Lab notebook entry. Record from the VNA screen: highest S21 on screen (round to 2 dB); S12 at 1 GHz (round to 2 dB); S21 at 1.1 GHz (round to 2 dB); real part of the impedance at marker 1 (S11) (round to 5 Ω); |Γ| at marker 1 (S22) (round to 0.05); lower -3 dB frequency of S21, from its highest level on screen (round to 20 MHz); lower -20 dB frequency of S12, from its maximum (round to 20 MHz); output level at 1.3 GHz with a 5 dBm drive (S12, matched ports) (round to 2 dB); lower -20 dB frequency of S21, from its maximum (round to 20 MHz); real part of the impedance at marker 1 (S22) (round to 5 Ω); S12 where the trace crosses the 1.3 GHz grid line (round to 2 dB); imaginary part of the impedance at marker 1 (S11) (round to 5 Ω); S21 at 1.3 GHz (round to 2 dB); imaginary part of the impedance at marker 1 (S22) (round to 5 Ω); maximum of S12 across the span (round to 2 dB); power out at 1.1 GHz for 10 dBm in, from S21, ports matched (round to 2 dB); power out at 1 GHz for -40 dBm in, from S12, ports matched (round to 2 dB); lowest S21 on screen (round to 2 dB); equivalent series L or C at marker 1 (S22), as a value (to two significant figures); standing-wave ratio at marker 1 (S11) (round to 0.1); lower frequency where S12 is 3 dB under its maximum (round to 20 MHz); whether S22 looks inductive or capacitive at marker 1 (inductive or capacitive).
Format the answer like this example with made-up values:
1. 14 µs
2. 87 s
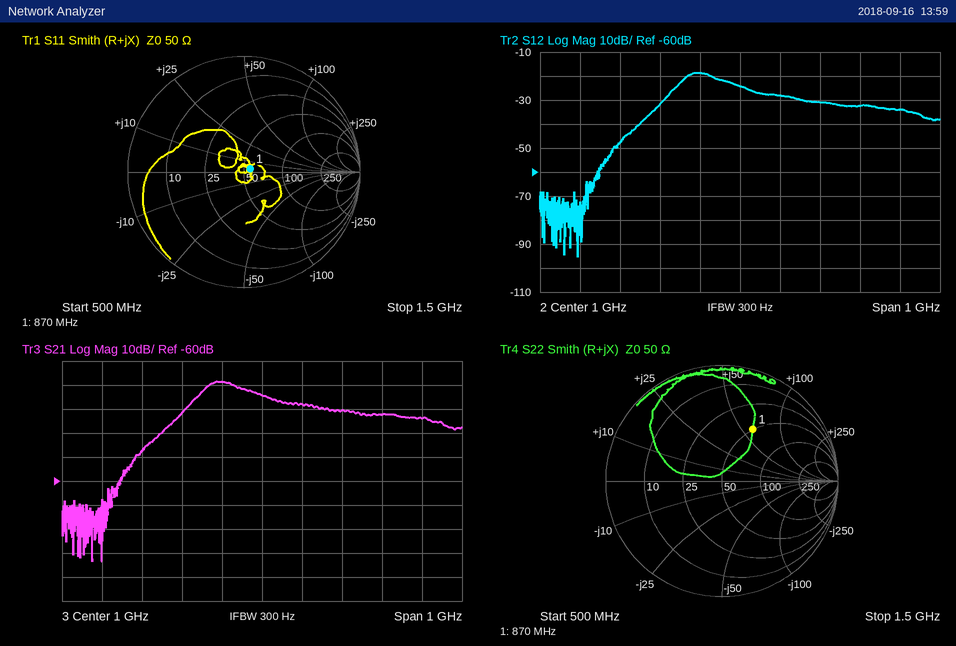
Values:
1. -18 dB
2. -24 dB
3. -28 dB
4. 55 Ω
5. 0.50
6. 860 MHz
7. 760 MHz
8. -28 dBm
9. 760 MHz
10. 50 Ω
11. -32 dB
12. +5 Ω
13. -32 dB
14. +60 Ω
15. -18 dB
16. -18 dBm
17. -64 dBm
18. -94 dB
19. 11 nH
20. 1.1
21. 860 MHz
22. inductive
